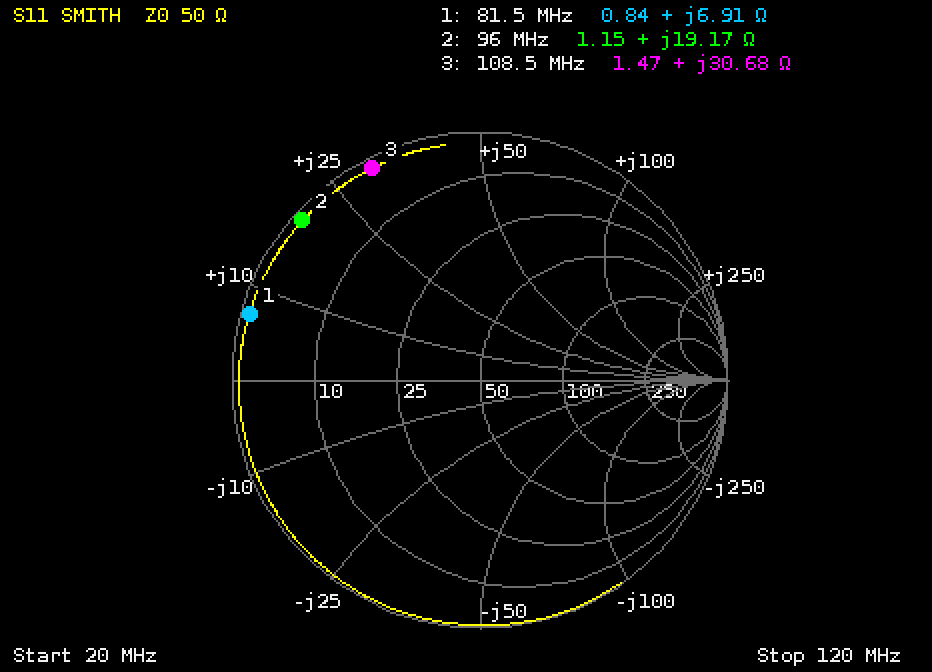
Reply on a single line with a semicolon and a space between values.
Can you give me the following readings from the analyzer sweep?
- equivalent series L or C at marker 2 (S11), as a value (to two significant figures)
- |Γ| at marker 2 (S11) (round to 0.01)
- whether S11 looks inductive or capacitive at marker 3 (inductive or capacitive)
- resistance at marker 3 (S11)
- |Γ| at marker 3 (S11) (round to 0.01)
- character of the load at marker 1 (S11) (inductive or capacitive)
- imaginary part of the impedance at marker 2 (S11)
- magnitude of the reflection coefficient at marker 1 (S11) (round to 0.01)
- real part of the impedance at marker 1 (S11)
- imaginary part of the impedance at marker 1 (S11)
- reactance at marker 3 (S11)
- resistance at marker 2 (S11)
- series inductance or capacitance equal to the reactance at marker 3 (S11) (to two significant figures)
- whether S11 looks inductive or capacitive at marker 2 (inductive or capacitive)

32 nH; 0.96; inductive; 1.47 Ω; 0.96; inductive; +19.17 Ω; 0.97; 0.84 Ω; +6.91 Ω; +30.68 Ω; 1.15 Ω; 45 nH; inductive
